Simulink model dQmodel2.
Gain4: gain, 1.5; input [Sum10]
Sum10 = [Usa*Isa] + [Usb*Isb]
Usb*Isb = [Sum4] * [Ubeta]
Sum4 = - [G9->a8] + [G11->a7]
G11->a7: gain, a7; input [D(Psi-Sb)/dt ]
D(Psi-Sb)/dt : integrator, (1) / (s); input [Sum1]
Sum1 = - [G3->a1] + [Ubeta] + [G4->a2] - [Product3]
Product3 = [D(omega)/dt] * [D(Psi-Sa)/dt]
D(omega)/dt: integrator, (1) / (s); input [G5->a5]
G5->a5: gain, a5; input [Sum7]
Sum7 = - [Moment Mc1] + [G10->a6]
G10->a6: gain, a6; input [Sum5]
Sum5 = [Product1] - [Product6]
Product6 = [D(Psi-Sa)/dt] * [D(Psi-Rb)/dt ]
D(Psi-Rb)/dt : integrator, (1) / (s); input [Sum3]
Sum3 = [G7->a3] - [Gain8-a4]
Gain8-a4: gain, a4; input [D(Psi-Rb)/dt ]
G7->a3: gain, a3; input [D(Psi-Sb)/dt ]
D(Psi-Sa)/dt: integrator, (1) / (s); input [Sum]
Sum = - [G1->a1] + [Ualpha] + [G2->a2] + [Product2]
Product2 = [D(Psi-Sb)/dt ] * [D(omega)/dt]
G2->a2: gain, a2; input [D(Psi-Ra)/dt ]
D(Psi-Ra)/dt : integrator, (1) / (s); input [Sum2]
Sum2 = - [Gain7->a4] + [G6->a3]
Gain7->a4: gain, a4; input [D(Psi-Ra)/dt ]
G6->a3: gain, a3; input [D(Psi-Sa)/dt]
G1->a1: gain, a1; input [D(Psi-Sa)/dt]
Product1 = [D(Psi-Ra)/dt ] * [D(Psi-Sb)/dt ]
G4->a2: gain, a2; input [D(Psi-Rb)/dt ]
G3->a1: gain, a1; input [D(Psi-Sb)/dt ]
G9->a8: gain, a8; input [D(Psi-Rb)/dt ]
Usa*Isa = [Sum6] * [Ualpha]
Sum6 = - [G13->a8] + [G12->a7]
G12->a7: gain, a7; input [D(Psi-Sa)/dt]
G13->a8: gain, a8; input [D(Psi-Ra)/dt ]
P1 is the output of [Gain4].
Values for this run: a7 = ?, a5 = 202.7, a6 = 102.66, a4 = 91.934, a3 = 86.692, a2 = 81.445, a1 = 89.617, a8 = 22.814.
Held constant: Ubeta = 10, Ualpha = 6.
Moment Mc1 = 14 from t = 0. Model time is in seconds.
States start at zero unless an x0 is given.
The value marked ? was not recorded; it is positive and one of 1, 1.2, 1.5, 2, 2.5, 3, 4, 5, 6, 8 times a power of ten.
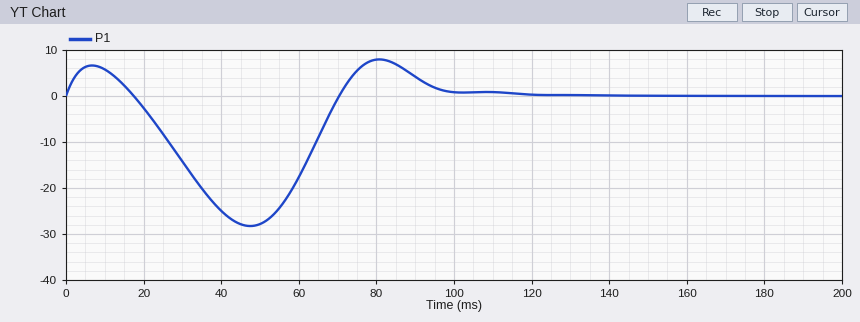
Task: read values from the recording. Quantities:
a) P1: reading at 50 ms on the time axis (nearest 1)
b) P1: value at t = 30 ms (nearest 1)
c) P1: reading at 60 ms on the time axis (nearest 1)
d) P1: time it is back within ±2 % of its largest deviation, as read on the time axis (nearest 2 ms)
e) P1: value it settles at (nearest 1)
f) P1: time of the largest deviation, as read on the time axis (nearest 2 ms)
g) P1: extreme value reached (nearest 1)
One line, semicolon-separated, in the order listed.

-28; -14; -18; 116 ms; 0; 48 ms; -28
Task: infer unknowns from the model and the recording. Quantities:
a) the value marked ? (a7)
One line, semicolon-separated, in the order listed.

12
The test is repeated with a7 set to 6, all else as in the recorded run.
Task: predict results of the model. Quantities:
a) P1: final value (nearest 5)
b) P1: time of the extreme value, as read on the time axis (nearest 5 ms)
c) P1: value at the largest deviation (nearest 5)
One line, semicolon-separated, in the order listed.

0; 40 ms; -35
